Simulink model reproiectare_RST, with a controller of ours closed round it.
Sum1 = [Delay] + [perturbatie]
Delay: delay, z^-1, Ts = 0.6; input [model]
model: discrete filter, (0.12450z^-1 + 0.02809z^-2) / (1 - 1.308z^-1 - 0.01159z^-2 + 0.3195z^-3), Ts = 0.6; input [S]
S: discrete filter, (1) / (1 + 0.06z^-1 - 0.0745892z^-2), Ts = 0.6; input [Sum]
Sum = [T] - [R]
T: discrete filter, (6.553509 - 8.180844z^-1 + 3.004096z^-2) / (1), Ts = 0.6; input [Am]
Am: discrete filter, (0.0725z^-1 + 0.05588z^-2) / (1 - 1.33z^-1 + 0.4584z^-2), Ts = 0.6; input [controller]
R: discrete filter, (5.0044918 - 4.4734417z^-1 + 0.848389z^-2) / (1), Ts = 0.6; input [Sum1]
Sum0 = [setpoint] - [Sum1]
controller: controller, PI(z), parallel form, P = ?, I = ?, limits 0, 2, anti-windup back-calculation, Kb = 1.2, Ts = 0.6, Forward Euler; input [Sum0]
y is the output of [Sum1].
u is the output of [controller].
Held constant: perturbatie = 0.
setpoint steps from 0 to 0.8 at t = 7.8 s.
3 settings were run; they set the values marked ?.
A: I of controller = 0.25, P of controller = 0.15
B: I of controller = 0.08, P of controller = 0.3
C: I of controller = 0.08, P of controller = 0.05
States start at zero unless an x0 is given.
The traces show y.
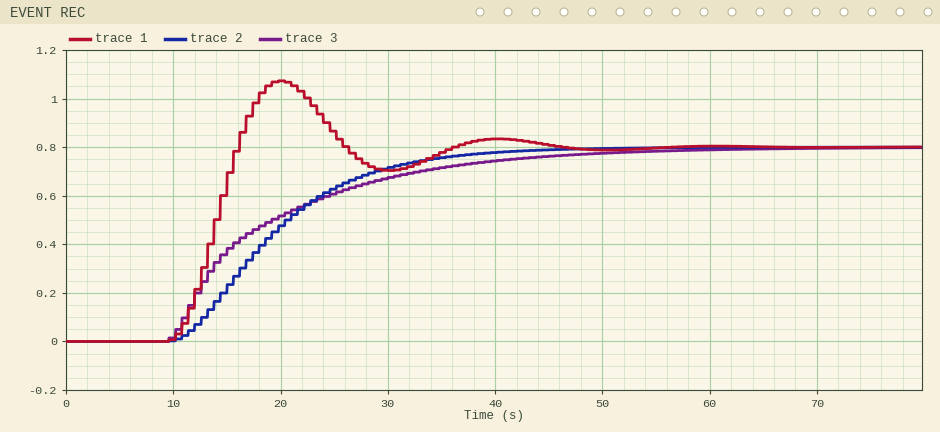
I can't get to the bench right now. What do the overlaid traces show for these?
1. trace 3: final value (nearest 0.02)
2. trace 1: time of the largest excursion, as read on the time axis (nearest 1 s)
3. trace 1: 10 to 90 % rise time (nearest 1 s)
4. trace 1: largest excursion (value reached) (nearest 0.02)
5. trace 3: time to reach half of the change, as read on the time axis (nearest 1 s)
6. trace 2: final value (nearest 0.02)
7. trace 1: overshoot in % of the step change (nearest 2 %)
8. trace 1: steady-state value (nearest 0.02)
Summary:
0.80
20 s
4 s
1.08
16 s
0.80
34 %
0.80
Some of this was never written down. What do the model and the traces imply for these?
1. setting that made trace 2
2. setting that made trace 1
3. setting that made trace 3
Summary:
C
A
B
